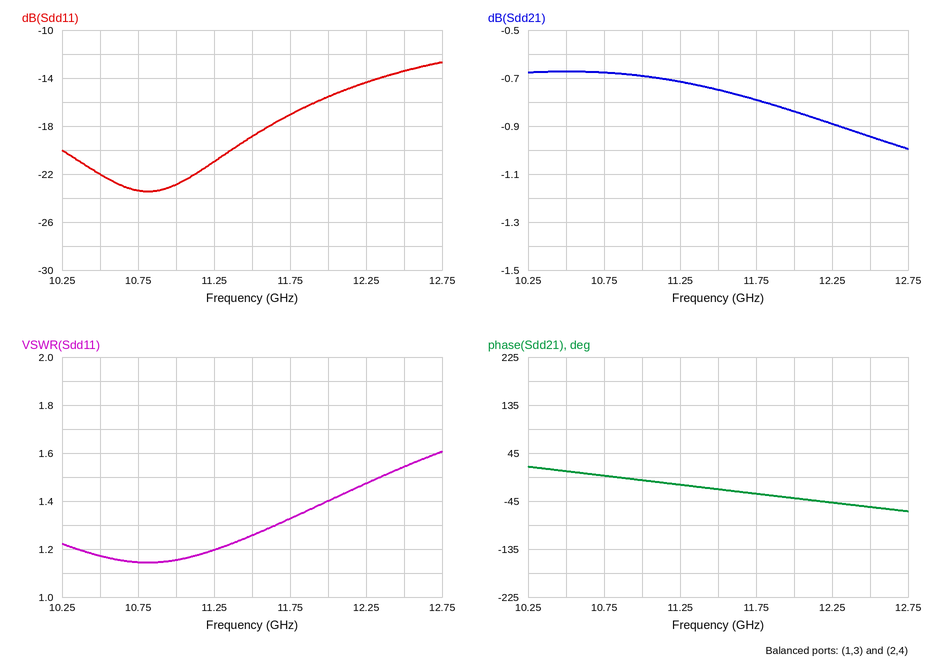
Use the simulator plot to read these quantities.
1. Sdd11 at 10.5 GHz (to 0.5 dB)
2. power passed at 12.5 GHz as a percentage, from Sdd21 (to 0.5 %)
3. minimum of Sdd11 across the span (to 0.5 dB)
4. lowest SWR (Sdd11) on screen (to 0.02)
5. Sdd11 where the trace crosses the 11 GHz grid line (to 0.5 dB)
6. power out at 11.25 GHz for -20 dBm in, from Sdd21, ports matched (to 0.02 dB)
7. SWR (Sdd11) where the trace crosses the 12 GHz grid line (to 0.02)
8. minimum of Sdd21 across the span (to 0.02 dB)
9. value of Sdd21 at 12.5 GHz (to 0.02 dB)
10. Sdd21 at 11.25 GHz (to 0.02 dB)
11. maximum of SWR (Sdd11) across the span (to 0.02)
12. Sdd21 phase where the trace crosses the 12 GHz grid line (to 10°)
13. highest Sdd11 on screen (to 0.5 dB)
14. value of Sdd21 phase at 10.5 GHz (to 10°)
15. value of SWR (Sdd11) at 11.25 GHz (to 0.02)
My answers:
-22.0 dB
80.5 %
-23.5 dB
1.14
-23.0 dB
-20.72 dBm
1.40
-1.00 dB
-0.94 dB
-0.72 dB
1.60
-40°
-12.5 dB
10°
1.20
